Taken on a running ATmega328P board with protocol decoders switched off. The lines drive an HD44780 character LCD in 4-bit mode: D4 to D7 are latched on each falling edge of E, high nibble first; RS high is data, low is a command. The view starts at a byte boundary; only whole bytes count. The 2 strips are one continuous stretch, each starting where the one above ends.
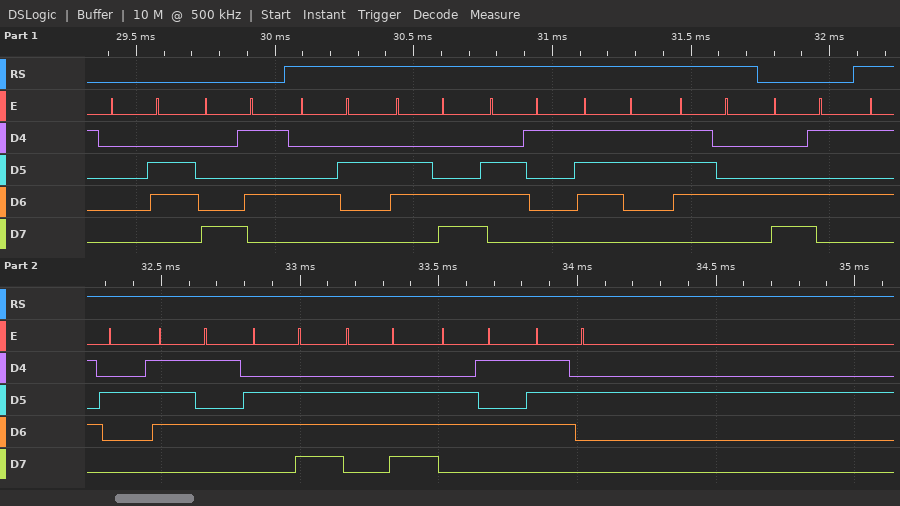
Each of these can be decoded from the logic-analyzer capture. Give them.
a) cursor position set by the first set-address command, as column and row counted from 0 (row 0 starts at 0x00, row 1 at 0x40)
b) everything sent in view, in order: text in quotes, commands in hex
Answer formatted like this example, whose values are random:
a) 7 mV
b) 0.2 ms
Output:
a) column 5, row 0
b) 0x06 0x85 "Blast" 0xC5 "Runner"
